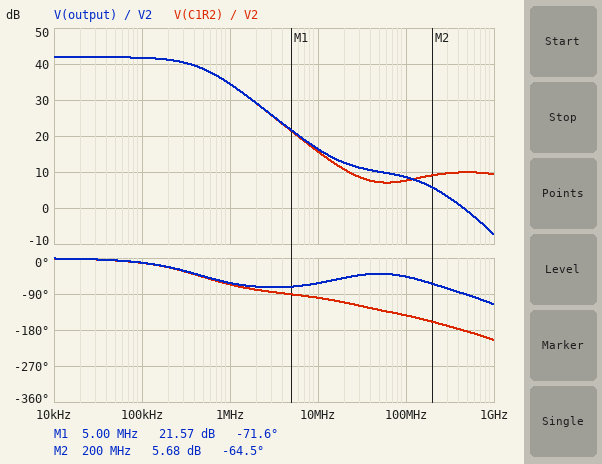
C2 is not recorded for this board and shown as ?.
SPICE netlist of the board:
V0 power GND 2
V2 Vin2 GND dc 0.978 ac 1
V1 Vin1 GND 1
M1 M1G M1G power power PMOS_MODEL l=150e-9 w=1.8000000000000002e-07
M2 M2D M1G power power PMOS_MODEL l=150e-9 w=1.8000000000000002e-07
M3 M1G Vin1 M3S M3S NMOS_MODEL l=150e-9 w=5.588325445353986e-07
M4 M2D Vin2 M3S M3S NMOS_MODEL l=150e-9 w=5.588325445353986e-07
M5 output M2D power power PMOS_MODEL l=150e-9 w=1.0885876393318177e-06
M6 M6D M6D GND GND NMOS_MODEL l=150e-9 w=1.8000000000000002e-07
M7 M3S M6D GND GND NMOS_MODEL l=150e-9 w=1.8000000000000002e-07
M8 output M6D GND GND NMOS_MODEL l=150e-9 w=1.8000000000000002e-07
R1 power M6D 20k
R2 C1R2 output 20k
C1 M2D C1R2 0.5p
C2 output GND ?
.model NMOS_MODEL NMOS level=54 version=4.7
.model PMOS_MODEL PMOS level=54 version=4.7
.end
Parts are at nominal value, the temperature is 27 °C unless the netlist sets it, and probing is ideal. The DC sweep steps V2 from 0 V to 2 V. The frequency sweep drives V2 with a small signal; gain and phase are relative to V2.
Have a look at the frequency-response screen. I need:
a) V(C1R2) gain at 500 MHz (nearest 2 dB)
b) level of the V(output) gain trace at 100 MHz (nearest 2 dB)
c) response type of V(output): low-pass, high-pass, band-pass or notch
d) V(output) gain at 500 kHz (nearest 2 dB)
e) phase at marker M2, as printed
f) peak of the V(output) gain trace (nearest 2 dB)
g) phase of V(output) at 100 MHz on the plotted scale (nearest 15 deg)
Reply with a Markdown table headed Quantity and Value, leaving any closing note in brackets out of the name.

| Quantity | Value |
|---|---|
| V(C1R2) gain at 500 MHz | 10 dB |
| level of the V(output) gain trace at 100 MHz | 8 dB |
| response type of V(output): low-pass, high-pass, band-pass or notch | low-pass |
| V(output) gain at 500 kHz | 38 dB |
| phase at marker M2, as printed | -64.5 deg |
| peak of the V(output) gain trace | 42 dB |
| phase of V(output) at 100 MHz on the plotted scale | -45 deg |
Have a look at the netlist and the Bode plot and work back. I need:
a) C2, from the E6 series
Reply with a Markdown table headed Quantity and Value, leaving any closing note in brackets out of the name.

| Quantity | Value |
|---|---|
| C2, from the E6 series | 330 fF |
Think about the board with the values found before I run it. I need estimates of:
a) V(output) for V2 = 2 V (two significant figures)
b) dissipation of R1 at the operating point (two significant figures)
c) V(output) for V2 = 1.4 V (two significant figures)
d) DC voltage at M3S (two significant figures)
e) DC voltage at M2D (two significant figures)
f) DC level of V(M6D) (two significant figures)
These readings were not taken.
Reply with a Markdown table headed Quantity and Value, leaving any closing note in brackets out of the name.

| Quantity | Value |
|---|---|
| V(output) for V2 = 2 V | 1.9 V |
| dissipation of R1 at the operating point | 59 µW |
| V(output) for V2 = 1.4 V | 1.9 V |
| DC voltage at M3S | 500 mV |
| DC voltage at M2D | 1.4 V |
| DC level of V(M6D) | 910 mV |
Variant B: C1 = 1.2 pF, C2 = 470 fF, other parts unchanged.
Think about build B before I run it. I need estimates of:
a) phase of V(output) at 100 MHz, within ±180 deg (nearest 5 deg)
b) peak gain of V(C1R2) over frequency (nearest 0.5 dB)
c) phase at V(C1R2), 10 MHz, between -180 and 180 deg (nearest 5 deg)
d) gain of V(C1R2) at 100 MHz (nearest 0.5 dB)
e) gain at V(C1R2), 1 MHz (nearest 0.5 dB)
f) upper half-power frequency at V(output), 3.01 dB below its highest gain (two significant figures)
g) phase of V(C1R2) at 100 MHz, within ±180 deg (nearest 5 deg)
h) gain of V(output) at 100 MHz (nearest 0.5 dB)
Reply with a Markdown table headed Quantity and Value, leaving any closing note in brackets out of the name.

| Quantity | Value |
|---|---|
| phase of V(output) at 100 MHz, within ±180 deg | -50 deg |
| peak gain of V(C1R2) over frequency | 42.0 dB |
| phase at V(C1R2), 10 MHz, between -180 and 180 deg | -110 deg |
| gain of V(C1R2) at 100 MHz | 8.0 dB |
| gain at V(C1R2), 1 MHz | 27.5 dB |
| upper half-power frequency at V(output), 3.01 dB below its highest gain | 200 kHz |
| phase of V(C1R2) at 100 MHz, within ±180 deg | -150 deg |
| gain of V(output) at 100 MHz | 7.5 dB |
